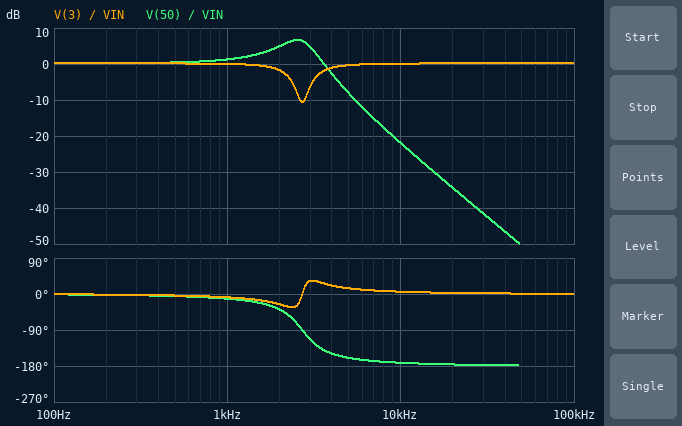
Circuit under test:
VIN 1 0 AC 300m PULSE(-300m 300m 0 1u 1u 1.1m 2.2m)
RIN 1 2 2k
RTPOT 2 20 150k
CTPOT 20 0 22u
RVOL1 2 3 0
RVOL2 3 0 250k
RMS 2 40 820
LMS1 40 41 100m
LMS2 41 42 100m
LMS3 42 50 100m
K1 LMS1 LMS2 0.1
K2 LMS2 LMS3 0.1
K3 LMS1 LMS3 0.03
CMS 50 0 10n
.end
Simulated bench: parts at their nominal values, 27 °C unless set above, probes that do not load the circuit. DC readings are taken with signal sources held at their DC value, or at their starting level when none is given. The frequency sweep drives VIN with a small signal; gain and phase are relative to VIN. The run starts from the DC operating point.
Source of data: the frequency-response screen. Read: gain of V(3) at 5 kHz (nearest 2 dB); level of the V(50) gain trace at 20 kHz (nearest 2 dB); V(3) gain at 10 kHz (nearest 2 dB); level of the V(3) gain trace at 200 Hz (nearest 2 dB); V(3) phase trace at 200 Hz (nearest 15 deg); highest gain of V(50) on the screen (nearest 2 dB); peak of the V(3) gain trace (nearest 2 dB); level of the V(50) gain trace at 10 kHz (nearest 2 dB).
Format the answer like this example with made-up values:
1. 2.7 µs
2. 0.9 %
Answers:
1. 0 dB
2. -34 dB
3. 0 dB
4. 0 dB
5. 0 deg
6. 6 dB
7. 0 dB
8. -22 dB
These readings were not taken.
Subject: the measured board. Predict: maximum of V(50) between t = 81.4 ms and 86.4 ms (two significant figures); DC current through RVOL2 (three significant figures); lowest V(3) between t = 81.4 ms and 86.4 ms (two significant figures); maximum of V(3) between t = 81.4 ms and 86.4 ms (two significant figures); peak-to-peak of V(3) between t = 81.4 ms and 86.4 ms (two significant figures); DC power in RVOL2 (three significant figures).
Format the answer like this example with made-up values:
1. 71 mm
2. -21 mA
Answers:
1. 580 mV
2. 1.23 µA
3. -380 mV
4. 370 mV
5. 750 mV
6. 376 nW
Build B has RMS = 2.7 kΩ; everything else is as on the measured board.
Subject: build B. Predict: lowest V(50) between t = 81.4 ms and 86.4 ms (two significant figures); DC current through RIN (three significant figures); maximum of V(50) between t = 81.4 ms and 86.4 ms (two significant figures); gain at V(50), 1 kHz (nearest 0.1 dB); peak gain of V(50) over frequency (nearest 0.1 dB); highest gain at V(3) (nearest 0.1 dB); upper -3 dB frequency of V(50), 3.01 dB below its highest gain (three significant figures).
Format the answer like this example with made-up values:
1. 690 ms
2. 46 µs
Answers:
1. -470 mV
2. 4.92 µA
3. 460 mV
4. 1.1 dB
5. 2.9 dB
6. 0.3 dB
7. 3.22 kHz
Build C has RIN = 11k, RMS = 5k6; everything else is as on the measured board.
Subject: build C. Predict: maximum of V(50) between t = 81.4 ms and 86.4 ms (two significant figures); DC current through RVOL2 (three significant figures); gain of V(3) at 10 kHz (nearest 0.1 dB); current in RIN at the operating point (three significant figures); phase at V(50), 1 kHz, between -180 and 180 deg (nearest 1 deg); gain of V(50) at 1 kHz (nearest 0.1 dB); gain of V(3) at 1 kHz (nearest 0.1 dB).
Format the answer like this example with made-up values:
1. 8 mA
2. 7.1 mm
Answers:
1. 370 mV
2. 1.66 µA
3. 0 dB
4. 10.5 µA
5. -57 deg
6. -1.1 dB
7. -1.7 dB
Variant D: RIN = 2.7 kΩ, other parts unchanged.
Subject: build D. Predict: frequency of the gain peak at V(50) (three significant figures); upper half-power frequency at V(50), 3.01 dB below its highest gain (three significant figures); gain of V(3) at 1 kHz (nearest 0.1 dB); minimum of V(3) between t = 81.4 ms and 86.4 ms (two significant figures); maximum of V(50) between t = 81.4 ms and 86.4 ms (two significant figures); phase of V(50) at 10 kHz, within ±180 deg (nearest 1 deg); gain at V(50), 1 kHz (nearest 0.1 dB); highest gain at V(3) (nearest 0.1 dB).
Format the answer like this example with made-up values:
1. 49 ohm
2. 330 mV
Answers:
1. 2.45 kHz
2. 3.19 kHz
3. -0.2 dB
4. -380 mV
5. 520 mV
6. -170 deg
7. 1.1 dB
8. 0.1 dB
